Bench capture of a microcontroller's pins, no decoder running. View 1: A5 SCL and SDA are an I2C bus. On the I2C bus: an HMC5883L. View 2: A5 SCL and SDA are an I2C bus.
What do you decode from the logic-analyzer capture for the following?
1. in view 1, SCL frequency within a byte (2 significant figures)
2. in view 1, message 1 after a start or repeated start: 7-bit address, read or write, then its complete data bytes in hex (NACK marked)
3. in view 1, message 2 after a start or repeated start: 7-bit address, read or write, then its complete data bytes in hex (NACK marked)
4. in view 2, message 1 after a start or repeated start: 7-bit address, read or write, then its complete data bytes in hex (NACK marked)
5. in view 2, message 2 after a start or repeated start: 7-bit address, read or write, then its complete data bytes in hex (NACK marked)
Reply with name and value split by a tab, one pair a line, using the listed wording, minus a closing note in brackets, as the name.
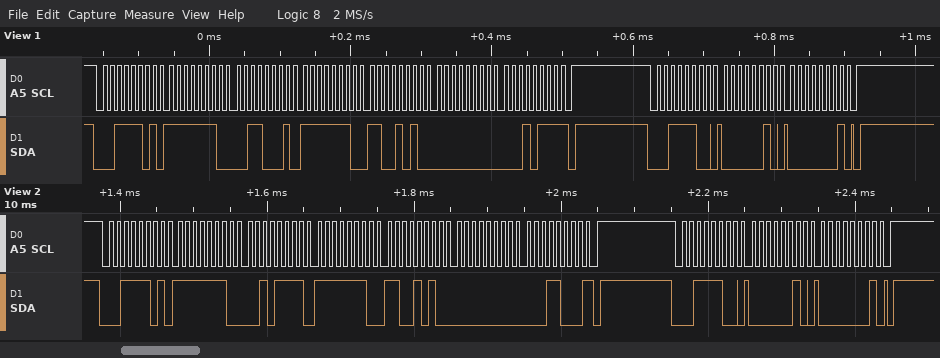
in view 1, SCL frequency within a byte	100 kHz
in view 1, message 1 after a start or repeated start: 7-bit address, read or write, then its complete data bytes in hex	0x1E read: FE 31 FE CA 00 17 NACK
in view 1, message 2 after a start or repeated start: 7-bit address, read or write, then its complete data bytes in hex	0x1E write: 02 01
in view 2, message 1 after a start or repeated start: 7-bit address, read or write, then its complete data bytes in hex	0x1E read: FE 2F FE CA 00 18 NACK
in view 2, message 2 after a start or repeated start: 7-bit address, read or write, then its complete data bytes in hex	0x1E write: 02 01
